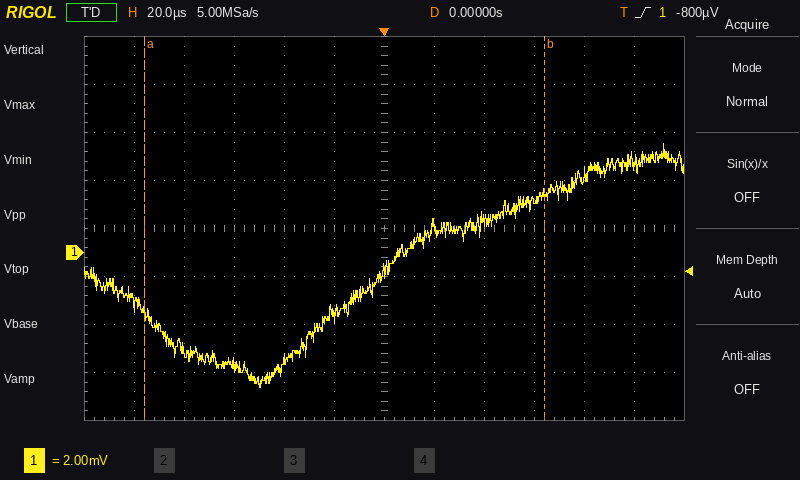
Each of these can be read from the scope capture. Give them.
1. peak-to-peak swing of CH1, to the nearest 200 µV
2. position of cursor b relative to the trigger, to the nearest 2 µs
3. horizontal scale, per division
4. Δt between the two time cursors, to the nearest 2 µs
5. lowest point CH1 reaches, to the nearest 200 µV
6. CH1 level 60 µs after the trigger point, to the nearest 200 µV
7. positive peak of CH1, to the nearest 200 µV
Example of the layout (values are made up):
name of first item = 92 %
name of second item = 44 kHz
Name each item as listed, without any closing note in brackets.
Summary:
peak-to-peak swing of CH1, to the nearest 200 µV = 10.2 mV
position of cursor b relative to the trigger, to the nearest 2 µs = +64 µs
horizontal scale, per division = 20 µs
Δt between the two time cursors, to the nearest 2 µs = 160 µs
lowest point CH1 reaches, to the nearest 200 µV = -5.6 mV
CH1 level 60 µs after the trigger point, to the nearest 200 µV = 2.2 mV
positive peak of CH1, to the nearest 200 µV = 4.6 mV
